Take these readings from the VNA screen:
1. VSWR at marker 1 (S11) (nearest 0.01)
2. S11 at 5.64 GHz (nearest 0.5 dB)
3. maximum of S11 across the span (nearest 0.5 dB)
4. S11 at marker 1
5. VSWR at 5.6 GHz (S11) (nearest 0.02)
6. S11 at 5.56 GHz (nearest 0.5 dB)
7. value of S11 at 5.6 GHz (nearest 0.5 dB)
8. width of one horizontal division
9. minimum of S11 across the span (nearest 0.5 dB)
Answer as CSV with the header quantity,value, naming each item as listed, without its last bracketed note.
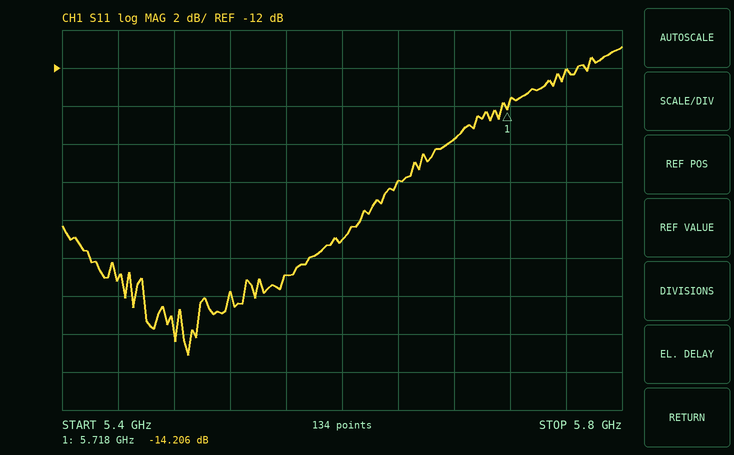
quantity,value
VSWR at marker 1 (S11),1.48
S11 at 5.64 GHz,-18.0 dB
maximum of S11 across the span,-11.0 dB
S11 at marker 1,-14.206 dB
VSWR at 5.6 GHz (S11),1.20
S11 at 5.56 GHz,-23.0 dB
value of S11 at 5.6 GHz,-21.0 dB
width of one horizontal division,40 MHz
minimum of S11 across the span,-27.0 dB
